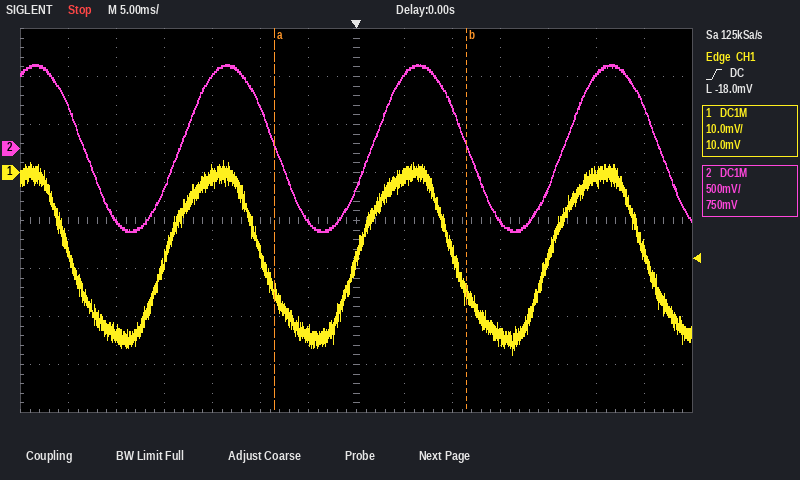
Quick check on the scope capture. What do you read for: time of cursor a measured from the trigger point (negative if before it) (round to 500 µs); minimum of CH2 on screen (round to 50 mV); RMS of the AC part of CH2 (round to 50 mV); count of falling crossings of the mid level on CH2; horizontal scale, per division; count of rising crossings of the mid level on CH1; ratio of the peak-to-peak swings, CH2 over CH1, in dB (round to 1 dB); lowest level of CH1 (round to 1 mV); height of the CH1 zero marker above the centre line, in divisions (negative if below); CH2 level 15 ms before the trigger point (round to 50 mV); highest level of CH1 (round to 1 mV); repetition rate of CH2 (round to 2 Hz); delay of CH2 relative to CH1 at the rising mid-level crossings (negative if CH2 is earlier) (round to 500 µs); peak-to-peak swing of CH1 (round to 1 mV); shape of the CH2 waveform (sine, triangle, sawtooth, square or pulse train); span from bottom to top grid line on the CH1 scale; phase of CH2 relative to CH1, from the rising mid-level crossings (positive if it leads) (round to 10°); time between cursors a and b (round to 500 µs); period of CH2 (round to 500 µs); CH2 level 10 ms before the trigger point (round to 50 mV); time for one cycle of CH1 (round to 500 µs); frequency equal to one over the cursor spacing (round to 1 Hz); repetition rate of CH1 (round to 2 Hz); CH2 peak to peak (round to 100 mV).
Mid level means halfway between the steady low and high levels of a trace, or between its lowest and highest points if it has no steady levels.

-8.5 ms
-850 mV
600 mV
4
5 ms
3
33 dB
-38 mV
+1.0 div
750 mV
2 mV
50 Hz
+1.5 ms
40 mV
sine
80 mV
-30°
20.0 ms
20.0 ms
450 mV
20.0 ms
50 Hz
50 Hz
1.70 V
